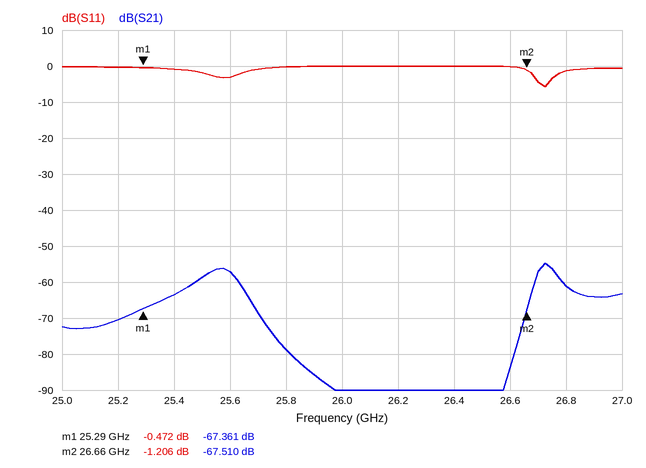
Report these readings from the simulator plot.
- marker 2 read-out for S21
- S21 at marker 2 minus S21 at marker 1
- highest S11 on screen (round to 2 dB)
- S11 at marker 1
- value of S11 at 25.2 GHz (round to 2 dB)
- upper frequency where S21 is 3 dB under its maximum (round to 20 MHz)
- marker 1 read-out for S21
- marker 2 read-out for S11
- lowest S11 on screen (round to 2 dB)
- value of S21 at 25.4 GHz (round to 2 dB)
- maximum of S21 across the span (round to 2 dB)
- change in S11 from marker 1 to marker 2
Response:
-67.510 dB
-0.149 dB
0 dB
-0.472 dB
0 dB
26.76 GHz
-67.361 dB
-1.206 dB
-6 dB
-64 dB
-54 dB
-0.734 dB
